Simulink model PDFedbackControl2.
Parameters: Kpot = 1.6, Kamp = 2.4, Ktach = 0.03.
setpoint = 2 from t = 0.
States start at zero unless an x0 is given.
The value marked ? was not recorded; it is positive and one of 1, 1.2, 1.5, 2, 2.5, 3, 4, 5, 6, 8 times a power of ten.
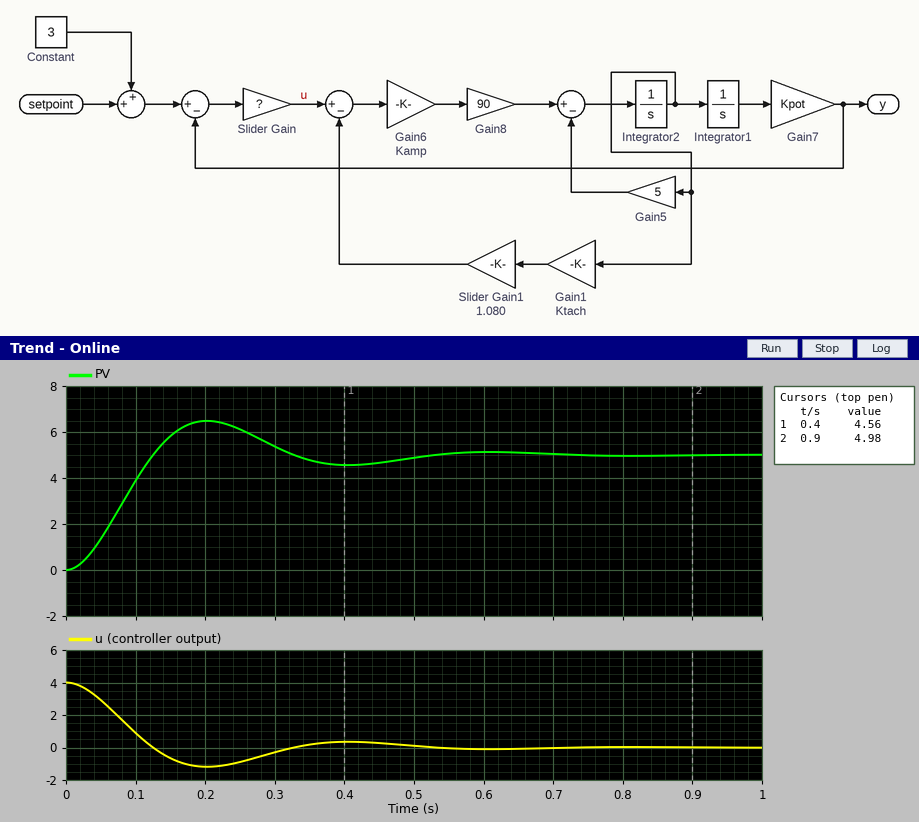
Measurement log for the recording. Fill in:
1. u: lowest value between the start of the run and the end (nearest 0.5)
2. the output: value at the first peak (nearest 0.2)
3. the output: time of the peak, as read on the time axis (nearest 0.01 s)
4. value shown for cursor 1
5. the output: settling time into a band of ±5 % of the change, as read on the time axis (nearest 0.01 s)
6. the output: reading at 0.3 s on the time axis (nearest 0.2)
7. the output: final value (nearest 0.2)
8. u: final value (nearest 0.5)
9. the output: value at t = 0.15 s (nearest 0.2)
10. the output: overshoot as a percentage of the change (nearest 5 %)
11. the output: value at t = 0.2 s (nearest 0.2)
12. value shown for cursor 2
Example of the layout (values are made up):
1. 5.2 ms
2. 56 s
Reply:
1. -1.0
2. 6.4
3. 0.20 s
4. 4.56
5. 0.47 s
6. 5.4
7. 5.0
8. 0.0
9. 5.8
10. 30 %
11. 6.4
12. 4.98
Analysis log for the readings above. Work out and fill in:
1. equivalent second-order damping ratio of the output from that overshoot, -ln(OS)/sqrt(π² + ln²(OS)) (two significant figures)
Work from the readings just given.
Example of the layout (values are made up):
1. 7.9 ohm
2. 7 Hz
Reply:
1. 0.36
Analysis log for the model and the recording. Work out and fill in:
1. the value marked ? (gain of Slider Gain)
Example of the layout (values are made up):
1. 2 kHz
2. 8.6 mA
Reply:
1. 0.8
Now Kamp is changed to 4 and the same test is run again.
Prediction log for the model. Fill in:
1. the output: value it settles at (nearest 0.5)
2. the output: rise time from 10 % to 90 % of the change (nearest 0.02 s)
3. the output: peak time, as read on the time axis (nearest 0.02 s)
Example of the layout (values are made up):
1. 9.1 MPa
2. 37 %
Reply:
1. 5.0
2. 0.06 s
3. 0.16 s
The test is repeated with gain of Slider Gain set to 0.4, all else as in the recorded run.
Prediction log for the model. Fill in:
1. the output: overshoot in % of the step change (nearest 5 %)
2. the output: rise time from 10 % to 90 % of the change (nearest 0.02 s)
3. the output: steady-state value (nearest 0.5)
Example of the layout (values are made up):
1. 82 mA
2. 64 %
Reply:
1. 15 %
2. 0.14 s
3. 5.0
